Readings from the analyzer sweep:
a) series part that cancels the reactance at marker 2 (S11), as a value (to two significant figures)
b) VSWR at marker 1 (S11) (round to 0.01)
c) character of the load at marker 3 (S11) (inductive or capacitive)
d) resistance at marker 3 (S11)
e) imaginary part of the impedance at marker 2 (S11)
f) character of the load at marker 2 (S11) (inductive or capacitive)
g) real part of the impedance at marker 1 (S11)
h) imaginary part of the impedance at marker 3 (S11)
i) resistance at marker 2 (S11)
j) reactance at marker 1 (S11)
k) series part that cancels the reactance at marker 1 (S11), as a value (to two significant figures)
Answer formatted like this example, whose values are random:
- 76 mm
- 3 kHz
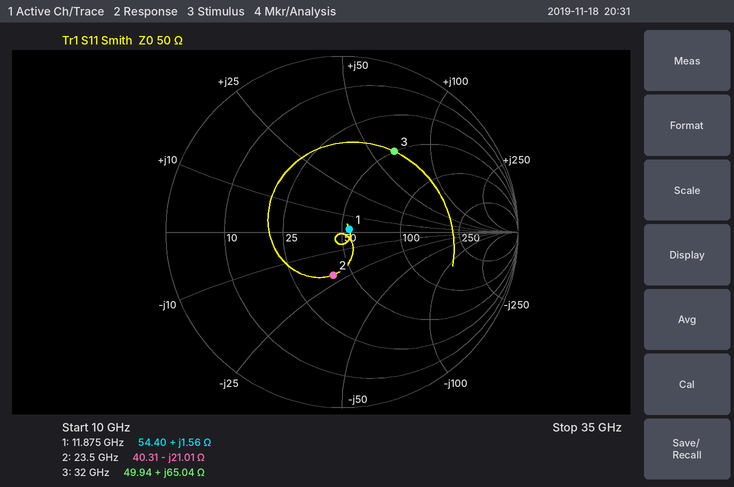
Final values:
- 140 pH
- 1.09
- inductive
- 49.94 Ω
- -21.01 Ω
- capacitive
- 54.40 Ω
- +65.04 Ω
- 40.31 Ω
- +1.56 Ω
- 8.6 pF
